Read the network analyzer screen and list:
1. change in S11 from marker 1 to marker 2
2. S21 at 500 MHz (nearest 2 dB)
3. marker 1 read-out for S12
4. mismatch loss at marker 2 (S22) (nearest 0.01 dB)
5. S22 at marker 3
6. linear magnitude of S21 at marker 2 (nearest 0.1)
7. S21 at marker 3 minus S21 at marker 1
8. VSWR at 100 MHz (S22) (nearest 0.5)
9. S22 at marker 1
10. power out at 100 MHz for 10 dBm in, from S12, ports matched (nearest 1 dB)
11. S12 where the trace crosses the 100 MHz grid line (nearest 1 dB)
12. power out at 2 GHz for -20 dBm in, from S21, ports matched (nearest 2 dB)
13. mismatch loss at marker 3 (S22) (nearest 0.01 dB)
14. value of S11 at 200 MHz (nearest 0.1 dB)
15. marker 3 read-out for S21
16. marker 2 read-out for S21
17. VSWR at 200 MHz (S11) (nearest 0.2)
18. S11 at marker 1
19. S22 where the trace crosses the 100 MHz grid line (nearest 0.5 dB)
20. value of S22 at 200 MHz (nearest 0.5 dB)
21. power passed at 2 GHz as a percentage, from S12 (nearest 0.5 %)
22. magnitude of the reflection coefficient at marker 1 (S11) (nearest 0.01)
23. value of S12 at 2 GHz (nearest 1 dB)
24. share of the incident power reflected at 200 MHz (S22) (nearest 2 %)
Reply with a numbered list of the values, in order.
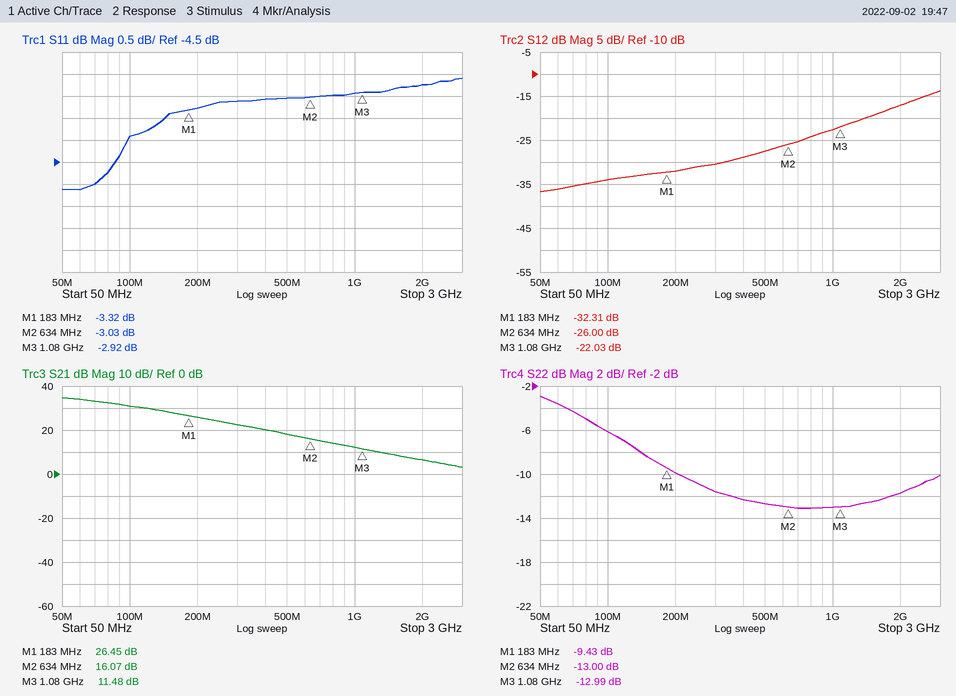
1. 0.29 dB
2. 18 dB
3. -32.31 dB
4. 0.22 dB
5. -12.99 dB
6. 6.4
7. -14.97 dB
8. 3.0
9. -9.43 dB
10. -24 dBm
11. -34 dB
12. -14 dBm
13. 0.22 dB
14. -3.3 dB
15. 11.48 dB
16. 16.07 dB
17. 5.4
18. -3.32 dB
19. -6.0 dB
20. -10.0 dB
21. 2.0 %
22. 0.68
23. -17 dB
24. 10 %
